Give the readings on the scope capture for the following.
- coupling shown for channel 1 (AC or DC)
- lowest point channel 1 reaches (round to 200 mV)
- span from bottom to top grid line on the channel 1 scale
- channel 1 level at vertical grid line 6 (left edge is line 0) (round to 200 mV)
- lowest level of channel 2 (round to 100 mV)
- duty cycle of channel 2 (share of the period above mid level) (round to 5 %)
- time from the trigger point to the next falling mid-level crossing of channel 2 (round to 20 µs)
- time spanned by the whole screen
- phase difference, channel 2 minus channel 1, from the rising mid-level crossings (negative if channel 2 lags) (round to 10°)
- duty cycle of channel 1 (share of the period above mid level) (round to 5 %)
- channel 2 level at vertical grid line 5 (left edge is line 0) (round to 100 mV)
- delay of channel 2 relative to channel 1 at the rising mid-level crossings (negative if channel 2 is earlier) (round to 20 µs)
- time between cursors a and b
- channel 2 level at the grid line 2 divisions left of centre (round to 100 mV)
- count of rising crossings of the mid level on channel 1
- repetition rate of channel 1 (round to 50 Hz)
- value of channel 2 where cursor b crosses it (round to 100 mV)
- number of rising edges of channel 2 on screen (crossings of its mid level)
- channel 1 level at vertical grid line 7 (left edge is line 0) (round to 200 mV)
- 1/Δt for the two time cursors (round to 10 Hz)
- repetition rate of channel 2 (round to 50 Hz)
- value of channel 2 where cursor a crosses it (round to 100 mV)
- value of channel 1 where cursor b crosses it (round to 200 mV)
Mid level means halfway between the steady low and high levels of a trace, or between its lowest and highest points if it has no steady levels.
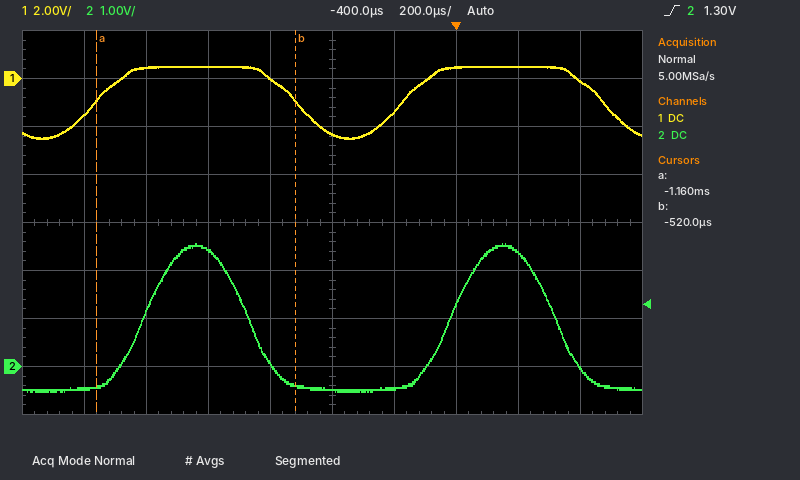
DC
-2.4 V
16 V
-1.4 V
-500 mV
35 %
320 µs
2 ms
-60°
65 %
-500 mV
+160 µs
640 µs
2.4 V
2
1.00 kHz
-400 mV
2
400 mV
1.56 kHz
1.00 kHz
-400 mV
-1.0 V
